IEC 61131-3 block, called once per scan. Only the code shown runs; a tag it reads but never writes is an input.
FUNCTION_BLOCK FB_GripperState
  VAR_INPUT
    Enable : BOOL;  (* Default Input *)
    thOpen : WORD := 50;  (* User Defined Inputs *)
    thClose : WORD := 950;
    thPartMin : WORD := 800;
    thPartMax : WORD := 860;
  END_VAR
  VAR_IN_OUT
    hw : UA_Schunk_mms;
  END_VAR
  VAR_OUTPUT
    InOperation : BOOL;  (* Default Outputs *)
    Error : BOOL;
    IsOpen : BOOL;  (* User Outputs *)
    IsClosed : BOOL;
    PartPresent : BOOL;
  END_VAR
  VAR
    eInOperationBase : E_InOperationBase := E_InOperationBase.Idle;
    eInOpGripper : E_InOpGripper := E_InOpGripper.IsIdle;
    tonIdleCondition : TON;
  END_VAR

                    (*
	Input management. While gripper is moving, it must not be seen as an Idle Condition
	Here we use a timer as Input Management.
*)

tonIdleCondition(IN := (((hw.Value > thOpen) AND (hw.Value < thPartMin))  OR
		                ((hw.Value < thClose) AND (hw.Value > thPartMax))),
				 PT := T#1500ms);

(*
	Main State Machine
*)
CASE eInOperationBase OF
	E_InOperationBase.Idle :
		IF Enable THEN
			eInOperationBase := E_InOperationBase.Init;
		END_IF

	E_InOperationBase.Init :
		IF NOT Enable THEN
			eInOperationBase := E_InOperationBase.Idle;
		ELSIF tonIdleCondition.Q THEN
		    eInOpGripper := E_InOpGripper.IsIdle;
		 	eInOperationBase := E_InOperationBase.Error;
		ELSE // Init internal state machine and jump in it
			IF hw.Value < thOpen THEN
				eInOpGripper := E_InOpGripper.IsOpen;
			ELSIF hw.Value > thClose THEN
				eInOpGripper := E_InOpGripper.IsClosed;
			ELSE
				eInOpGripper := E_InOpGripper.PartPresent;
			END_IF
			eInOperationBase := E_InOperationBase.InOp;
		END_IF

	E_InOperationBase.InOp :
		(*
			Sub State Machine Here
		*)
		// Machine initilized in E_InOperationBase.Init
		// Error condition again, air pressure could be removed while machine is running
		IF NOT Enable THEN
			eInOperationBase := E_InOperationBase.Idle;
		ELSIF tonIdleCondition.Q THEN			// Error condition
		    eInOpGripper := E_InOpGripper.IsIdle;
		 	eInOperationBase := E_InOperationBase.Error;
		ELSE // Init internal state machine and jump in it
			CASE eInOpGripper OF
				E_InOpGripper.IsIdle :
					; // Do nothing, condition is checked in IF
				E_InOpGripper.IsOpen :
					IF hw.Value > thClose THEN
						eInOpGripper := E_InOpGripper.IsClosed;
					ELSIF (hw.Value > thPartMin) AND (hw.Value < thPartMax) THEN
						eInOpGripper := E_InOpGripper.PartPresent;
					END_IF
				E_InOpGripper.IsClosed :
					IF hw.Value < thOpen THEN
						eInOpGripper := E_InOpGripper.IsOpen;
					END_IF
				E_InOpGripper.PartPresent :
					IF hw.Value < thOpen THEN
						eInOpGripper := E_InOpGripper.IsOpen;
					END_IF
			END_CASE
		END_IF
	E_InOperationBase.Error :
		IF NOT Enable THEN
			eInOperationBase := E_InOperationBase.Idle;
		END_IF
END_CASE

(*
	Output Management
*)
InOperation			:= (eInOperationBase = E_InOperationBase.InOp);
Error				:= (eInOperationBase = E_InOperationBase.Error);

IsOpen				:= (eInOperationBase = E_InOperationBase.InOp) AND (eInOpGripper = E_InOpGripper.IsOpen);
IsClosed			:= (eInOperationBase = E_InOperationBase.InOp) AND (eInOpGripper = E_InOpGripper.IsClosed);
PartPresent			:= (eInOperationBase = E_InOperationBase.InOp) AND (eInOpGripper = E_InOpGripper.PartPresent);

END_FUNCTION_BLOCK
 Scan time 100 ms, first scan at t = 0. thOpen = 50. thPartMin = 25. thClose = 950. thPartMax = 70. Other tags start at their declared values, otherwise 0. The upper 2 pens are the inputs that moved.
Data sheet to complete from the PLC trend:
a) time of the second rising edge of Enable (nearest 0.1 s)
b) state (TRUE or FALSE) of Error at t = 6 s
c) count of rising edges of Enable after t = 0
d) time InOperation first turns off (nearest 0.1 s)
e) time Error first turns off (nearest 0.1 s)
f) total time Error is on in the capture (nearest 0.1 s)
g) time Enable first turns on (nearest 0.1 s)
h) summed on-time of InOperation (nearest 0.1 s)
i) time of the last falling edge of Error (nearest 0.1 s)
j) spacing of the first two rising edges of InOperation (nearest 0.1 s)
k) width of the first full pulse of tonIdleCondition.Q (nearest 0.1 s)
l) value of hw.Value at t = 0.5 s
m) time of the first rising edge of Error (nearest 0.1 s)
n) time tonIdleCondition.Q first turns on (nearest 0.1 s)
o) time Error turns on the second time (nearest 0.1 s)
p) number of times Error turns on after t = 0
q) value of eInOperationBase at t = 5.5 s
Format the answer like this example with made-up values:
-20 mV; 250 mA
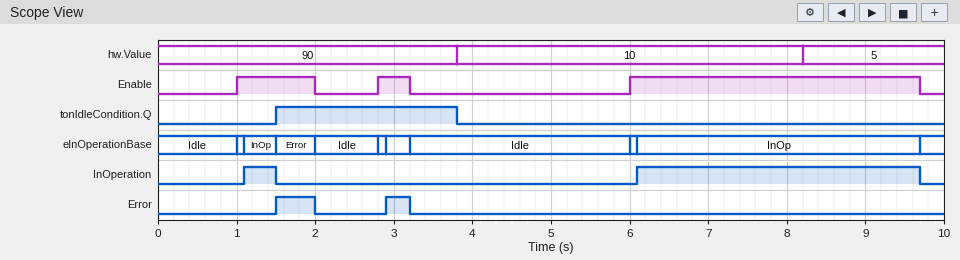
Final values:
2.8 s; FALSE; 3; 1.5 s; 2.0 s; 0.8 s; 1.0 s; 4.0 s; 3.2 s; 5.0 s; 2.3 s; 90; 1.5 s; 1.5 s; 2.9 s; 2; Idle
